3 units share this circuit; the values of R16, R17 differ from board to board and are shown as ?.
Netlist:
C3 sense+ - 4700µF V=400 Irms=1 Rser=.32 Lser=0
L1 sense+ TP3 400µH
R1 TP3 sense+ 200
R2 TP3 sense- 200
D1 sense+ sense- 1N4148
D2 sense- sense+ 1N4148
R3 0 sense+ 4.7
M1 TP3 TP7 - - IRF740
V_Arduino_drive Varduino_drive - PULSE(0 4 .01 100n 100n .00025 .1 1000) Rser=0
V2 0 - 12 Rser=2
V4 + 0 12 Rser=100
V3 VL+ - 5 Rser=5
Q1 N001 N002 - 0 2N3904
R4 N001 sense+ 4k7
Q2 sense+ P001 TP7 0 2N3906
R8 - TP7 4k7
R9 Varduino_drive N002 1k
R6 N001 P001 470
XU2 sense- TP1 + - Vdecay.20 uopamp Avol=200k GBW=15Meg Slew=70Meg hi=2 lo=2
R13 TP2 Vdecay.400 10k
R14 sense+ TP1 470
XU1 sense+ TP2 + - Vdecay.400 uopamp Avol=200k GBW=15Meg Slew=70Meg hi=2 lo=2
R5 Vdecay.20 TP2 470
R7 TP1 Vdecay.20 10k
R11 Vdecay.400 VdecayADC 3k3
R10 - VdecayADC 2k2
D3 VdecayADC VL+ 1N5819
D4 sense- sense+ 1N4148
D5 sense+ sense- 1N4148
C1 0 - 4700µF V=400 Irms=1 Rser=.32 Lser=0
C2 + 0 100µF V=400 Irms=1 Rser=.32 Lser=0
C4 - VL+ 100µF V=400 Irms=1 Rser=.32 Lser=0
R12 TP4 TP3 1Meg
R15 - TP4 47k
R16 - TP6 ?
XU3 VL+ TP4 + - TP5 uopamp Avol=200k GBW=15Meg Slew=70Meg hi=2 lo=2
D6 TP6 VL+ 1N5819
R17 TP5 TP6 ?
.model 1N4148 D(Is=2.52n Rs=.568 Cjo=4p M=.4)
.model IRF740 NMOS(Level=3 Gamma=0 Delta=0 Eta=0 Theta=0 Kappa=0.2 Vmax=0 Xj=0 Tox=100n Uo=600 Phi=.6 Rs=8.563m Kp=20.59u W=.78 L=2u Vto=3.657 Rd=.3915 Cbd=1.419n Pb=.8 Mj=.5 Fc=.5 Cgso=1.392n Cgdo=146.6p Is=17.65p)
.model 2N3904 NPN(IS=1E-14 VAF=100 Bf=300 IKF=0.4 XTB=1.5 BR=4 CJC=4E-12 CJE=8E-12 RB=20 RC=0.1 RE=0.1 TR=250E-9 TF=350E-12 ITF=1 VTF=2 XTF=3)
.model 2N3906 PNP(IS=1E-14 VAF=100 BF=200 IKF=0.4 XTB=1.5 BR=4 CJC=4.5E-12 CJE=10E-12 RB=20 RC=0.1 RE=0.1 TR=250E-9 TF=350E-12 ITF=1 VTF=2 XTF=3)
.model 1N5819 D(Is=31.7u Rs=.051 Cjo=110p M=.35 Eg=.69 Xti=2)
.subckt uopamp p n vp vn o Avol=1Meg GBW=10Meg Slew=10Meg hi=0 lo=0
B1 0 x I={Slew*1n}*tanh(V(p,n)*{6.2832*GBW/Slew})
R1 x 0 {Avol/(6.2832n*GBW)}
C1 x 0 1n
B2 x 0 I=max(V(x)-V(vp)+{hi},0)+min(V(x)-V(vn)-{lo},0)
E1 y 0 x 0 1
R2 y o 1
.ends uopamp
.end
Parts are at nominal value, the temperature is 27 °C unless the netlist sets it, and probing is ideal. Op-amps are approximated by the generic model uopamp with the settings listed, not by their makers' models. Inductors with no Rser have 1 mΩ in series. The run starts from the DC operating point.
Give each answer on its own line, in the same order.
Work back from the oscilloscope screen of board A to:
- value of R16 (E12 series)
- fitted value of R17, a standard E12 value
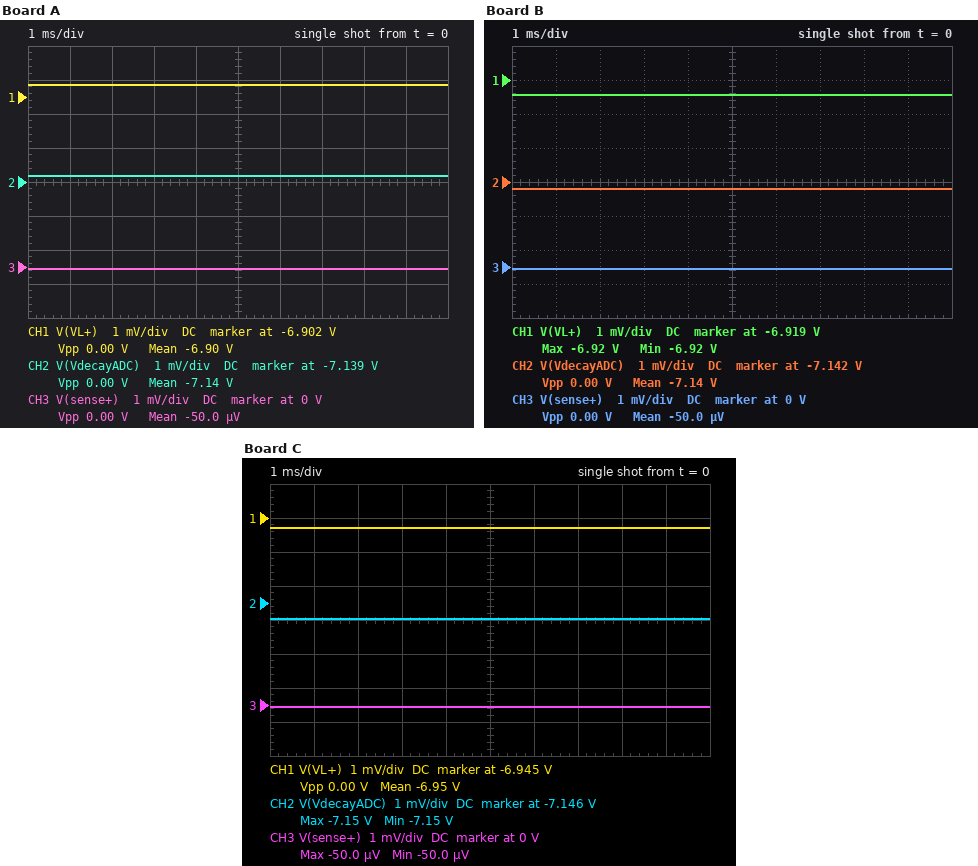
6.8 kΩ
1.2 kΩ
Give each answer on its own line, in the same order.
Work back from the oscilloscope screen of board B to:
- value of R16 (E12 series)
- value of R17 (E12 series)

12 kΩ
1.5 kΩ
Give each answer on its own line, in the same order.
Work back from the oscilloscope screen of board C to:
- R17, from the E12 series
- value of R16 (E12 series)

2.2 kΩ
8.2 kΩ
